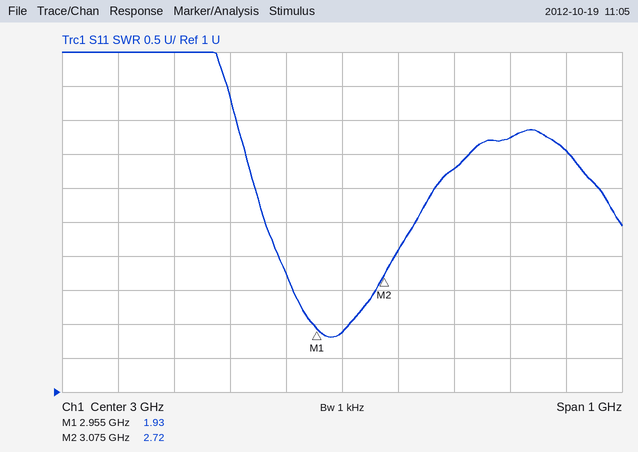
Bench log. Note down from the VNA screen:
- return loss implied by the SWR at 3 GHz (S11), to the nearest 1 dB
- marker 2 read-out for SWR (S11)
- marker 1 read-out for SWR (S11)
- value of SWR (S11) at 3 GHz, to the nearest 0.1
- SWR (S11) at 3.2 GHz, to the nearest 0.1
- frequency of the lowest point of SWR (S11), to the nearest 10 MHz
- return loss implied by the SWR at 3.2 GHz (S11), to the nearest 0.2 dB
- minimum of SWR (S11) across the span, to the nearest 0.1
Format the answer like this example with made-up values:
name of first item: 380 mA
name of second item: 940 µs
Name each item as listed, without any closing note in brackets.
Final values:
return loss implied by the SWR at 3 GHz (S11), to the nearest 1 dB: 10 dB
marker 2 read-out for SWR: 2.72
marker 1 read-out for SWR: 1.93
value of SWR (S11) at 3 GHz, to the nearest 0.1: 1.9
SWR (S11) at 3.2 GHz, to the nearest 0.1: 4.3
frequency of the lowest point of SWR (S11), to the nearest 10 MHz: 2.98 GHz
return loss implied by the SWR at 3.2 GHz (S11), to the nearest 0.2 dB: 4.2 dB
minimum of SWR (S11) across the span, to the nearest 0.1: 1.8
